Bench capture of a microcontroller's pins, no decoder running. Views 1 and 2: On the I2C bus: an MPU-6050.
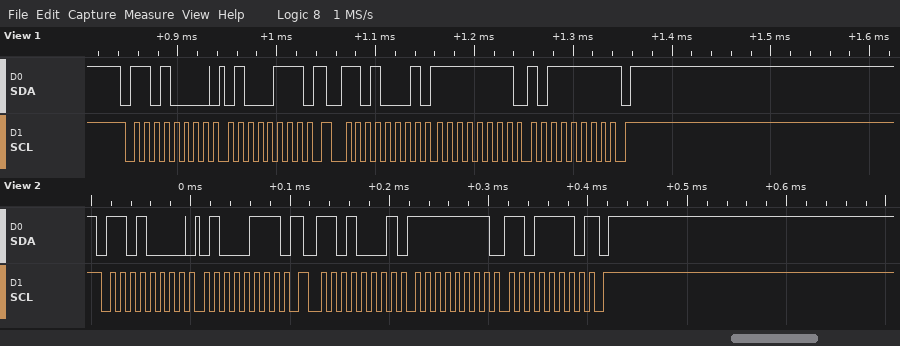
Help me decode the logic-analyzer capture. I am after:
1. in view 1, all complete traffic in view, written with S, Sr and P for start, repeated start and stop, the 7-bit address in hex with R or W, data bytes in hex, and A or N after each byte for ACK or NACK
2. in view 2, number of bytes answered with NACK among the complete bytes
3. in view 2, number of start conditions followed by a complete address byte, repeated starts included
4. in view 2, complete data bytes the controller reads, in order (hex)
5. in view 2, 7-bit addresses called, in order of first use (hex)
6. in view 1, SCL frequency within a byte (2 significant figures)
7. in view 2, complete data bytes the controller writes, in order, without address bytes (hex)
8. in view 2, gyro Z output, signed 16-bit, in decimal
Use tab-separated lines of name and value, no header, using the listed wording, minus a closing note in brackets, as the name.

in view 1, all complete traffic in view, written with S, Sr and P for start, repeated start and stop, the 7-bit address in hex with R or W, data bytes in hex, and A or N after each byte for ACK or NACK	S 68W A 47 A Sr 68R A FF A BF N P
in view 2, number of bytes answered with NACK among the complete bytes	1
in view 2, number of start conditions followed by a complete address byte, repeated starts included	2
in view 2, complete data bytes the controller reads, in order	FF DE
in view 2, 7-bit addresses called, in order of first use	0x68
in view 1, SCL frequency within a byte	100 kHz
in view 2, complete data bytes the controller writes, in order, without address bytes	47
in view 2, gyro Z output, signed 16-bit, in decimal	-34
